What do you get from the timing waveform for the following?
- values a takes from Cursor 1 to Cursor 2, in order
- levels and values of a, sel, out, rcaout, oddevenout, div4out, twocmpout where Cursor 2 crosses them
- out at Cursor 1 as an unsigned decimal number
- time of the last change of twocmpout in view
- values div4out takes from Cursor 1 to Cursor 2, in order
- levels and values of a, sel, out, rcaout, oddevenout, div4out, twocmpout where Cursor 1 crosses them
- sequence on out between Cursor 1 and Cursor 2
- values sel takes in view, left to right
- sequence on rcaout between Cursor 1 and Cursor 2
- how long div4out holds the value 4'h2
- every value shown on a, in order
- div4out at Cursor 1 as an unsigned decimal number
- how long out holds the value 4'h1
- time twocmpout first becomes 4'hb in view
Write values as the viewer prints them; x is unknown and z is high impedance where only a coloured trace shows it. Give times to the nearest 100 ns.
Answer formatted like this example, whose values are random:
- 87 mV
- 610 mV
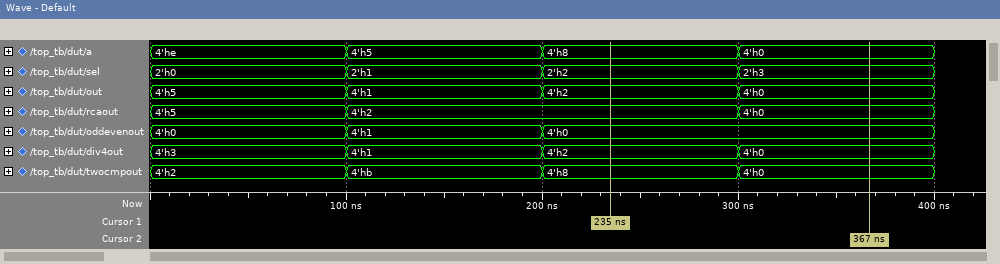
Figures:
- 4'h8, 4'h0
- a=4'h0, sel=2'h3, out=4'h0, rcaout=4'h0, oddevenout=4'h0, div4out=4'h0, twocmpout=4'h0
- 2
- 300 ns
- 4'h2, 4'h0
- a=4'h8, sel=2'h2, out=4'h2, rcaout=4'h2, oddevenout=4'h0, div4out=4'h2, twocmpout=4'h8
- 4'h2, 4'h0
- 2'h0, 2'h1, 2'h2, 2'h3
- 4'h2, 4'h0
- 100 ns
- 4'he, 4'h5, 4'h8, 4'h0
- 2
- 100 ns
- 100 ns
